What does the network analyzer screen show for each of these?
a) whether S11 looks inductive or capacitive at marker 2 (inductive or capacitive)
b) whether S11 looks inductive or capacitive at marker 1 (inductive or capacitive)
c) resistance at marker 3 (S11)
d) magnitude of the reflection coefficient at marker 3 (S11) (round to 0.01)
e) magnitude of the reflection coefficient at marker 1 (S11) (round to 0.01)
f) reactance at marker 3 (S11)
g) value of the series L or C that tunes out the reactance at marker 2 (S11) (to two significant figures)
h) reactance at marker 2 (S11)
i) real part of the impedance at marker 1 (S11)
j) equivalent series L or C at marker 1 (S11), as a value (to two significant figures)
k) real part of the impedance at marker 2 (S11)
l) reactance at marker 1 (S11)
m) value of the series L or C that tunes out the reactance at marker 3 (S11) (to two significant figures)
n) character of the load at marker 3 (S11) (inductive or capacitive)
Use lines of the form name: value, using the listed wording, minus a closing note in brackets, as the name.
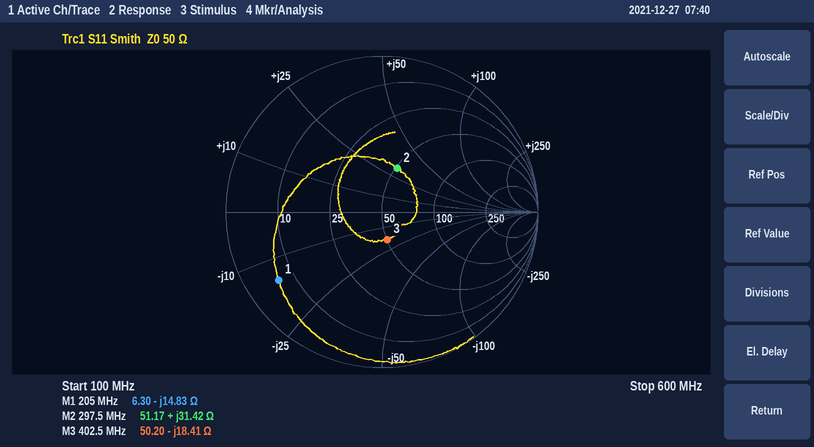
whether S11 looks inductive or capacitive at marker 2: inductive
whether S11 looks inductive or capacitive at marker 1: capacitive
resistance at marker 3: 50.20 Ω
magnitude of the reflection coefficient at marker 3 (S11): 0.18
magnitude of the reflection coefficient at marker 1 (S11): 0.79
reactance at marker 3: -18.41 Ω
value of the series L or C that tunes out the reactance at marker 2 (S11): 17 pF
reactance at marker 2: +31.42 Ω
real part of the impedance at marker 1: 6.30 Ω
equivalent series L or C at marker 1 (S11), as a value: 52 pF
real part of the impedance at marker 2: 51.17 Ω
reactance at marker 1: -14.83 Ω
value of the series L or C that tunes out the reactance at marker 3 (S11): 7.3 nH
character of the load at marker 3 (S11): capacitive
